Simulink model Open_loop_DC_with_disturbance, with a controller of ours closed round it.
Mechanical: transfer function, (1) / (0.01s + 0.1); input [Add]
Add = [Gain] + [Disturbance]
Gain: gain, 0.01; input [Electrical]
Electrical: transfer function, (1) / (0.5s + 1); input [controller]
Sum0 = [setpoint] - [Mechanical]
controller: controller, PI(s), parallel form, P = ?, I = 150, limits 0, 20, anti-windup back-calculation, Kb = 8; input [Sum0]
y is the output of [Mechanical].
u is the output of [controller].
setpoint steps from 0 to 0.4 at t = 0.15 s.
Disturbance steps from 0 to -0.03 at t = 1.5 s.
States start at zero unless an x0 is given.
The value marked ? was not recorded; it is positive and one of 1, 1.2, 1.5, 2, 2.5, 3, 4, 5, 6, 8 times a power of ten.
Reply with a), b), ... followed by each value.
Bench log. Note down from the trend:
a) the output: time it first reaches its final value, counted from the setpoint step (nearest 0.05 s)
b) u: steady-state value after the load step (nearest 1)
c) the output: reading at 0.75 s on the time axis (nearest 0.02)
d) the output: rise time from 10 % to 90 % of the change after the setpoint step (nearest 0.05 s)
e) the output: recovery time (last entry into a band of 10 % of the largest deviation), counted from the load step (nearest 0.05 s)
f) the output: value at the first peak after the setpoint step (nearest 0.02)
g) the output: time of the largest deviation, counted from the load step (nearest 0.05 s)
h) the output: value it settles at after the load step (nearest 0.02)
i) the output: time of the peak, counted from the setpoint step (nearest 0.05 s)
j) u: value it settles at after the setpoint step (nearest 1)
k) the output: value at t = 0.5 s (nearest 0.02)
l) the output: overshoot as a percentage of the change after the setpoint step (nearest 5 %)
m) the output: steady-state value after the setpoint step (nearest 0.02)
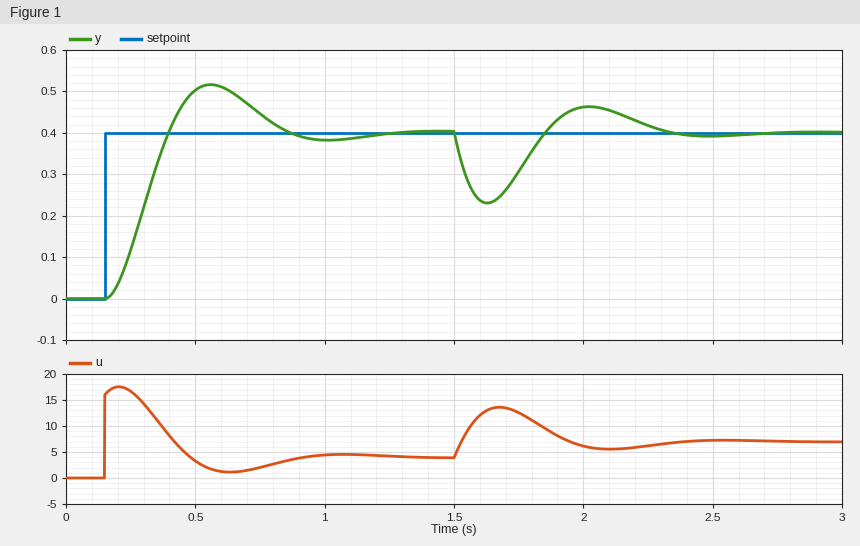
a) 0.25 s
b) 7
c) 0.44
d) 0.15 s
e) 0.75 s
f) 0.52
g) 0.15 s
h) 0.40
i) 0.40 s
j) 4
k) 0.50
l) 30 %
m) 0.40
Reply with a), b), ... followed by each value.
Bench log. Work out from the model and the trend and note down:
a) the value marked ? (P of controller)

a) 40
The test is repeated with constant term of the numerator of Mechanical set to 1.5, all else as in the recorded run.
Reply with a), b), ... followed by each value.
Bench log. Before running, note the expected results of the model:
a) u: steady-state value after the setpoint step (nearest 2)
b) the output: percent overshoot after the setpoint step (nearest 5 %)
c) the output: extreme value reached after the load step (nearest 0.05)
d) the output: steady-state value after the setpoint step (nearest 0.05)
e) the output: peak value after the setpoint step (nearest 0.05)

a) 2
b) 35 %
c) 0.15
d) 0.40
e) 0.55
